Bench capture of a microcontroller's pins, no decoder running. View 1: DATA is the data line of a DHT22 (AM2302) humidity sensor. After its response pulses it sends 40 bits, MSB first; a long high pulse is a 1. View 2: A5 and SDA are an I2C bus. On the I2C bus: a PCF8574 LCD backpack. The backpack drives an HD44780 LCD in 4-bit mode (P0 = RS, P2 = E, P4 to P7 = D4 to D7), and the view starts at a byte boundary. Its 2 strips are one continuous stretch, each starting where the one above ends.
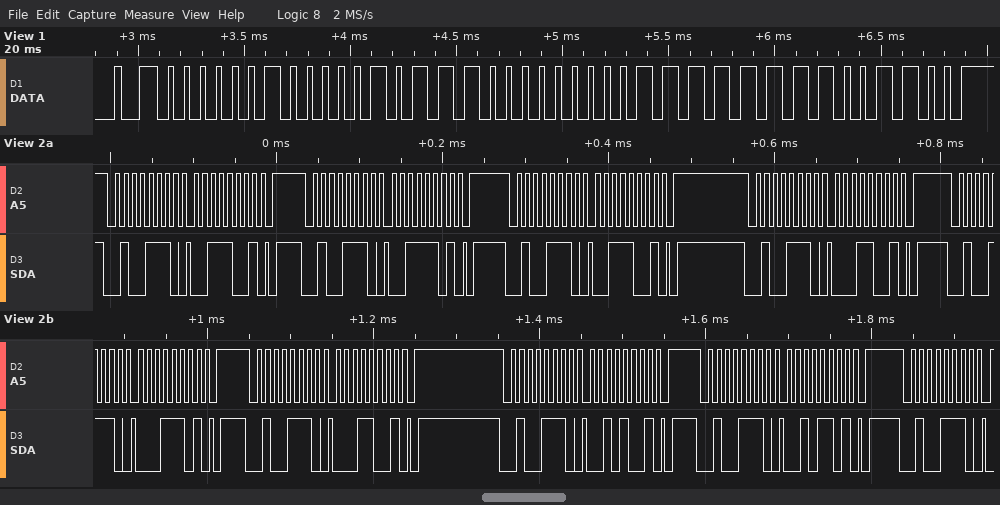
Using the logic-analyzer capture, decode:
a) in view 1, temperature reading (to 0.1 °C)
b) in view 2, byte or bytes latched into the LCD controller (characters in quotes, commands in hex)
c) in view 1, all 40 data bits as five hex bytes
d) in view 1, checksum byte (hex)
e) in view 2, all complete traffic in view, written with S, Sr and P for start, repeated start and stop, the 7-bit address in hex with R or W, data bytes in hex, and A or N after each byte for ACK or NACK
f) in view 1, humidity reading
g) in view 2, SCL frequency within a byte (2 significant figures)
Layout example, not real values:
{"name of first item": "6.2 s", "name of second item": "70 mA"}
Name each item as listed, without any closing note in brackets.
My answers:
{"in view 1, temperature reading": "-6.3 °C", "in view 2, byte or bytes latched into the LCD controller": "'1'", "in view 1, all 40 data bits as five hex bytes": "02 0B 80 3F CC", "in view 1, checksum byte": "0xCC", "in view 2, all complete traffic in view, written with S, Sr and P for start, repeated start and stop, the 7-bit address in hex with R or W, data bytes in hex, and A or N after each byte for ACK or NACK": "S 27W A 39 A P S 27W A 3D A P S 27W A 39 A P S 27W A 19 A P S 27W A 1D A P S 27W A 19 A P S 27W A 29 A P S 27W A 2D A P S 27W A", "in view 1, humidity reading": "52.3 %", "in view 2, SCL frequency within a byte": "100 kHz"}
